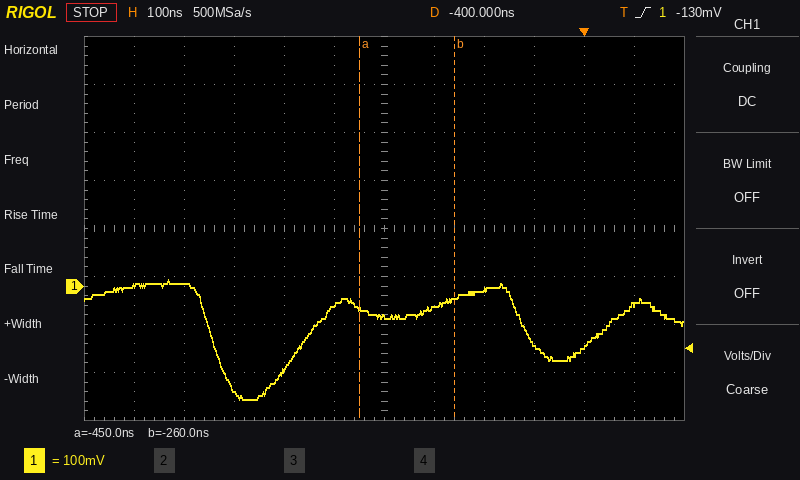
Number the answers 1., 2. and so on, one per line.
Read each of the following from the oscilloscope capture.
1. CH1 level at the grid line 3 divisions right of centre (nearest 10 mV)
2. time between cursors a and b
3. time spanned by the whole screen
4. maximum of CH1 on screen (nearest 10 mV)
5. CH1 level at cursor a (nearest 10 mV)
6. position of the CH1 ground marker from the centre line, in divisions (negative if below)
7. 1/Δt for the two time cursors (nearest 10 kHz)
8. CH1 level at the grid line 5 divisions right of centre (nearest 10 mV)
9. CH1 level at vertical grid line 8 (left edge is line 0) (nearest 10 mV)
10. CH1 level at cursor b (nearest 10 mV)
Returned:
1. -120 mV
2. 190 ns
3. 1.2 µs
4. 10 mV
5. -50 mV
6. -1.2 div
7. 5.26 MHz
8. -40 mV
9. -10 mV
10. -30 mV
